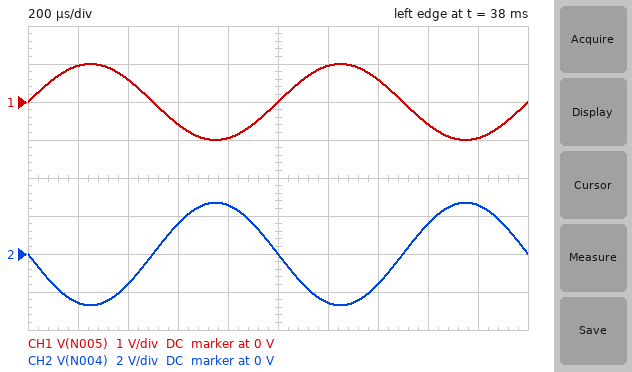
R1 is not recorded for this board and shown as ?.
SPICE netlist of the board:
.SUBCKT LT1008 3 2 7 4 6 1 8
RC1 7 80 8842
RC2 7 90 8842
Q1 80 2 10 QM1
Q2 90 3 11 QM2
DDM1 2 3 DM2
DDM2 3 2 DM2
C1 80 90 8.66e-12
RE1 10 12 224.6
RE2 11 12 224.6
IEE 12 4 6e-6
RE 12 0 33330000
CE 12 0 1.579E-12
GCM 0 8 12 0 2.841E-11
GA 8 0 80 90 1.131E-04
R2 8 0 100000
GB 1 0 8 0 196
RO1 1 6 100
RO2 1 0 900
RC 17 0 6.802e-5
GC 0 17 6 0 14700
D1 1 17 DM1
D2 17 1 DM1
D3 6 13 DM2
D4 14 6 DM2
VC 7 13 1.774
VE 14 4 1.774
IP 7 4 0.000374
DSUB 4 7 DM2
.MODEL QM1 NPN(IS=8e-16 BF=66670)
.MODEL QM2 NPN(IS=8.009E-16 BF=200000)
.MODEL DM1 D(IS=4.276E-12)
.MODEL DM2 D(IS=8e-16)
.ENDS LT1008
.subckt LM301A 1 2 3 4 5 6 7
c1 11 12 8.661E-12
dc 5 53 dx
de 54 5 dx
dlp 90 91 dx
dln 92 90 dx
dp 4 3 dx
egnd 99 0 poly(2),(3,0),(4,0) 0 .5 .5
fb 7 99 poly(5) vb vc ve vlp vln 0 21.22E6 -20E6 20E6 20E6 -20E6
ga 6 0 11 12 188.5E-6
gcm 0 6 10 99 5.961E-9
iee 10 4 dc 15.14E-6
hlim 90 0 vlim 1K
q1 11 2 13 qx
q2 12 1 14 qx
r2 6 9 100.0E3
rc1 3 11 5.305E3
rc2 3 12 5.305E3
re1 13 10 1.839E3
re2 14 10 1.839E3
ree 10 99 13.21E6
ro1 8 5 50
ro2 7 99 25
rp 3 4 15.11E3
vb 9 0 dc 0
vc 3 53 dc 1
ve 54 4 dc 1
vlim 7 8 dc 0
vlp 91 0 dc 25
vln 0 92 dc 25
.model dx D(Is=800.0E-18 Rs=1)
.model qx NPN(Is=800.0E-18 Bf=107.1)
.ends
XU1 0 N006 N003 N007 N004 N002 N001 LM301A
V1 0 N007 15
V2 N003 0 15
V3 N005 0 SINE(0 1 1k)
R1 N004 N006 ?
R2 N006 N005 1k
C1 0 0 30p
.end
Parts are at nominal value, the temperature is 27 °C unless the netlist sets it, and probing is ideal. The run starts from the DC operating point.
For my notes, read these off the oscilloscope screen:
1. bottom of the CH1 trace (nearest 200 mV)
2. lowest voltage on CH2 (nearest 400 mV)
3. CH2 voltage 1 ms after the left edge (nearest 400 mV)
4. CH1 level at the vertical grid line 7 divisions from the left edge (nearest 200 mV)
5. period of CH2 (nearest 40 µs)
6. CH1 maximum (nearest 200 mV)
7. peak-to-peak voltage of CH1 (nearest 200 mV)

-1.0 V
-2.8 V
0 V
600 mV
1.00 ms
1.0 V
2.0 V
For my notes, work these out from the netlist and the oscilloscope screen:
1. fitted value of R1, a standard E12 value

2.7 kΩ
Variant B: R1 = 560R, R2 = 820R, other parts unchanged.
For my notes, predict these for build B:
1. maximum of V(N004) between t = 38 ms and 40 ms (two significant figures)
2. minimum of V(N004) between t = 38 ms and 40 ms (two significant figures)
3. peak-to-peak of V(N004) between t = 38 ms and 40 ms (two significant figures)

680 mV
-680 mV
1.4 V
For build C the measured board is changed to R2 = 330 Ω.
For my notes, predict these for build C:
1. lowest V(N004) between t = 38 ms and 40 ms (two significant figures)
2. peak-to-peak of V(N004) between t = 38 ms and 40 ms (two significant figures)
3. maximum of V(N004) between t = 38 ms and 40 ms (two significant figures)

-8.2 V
16 V
8.2 V
